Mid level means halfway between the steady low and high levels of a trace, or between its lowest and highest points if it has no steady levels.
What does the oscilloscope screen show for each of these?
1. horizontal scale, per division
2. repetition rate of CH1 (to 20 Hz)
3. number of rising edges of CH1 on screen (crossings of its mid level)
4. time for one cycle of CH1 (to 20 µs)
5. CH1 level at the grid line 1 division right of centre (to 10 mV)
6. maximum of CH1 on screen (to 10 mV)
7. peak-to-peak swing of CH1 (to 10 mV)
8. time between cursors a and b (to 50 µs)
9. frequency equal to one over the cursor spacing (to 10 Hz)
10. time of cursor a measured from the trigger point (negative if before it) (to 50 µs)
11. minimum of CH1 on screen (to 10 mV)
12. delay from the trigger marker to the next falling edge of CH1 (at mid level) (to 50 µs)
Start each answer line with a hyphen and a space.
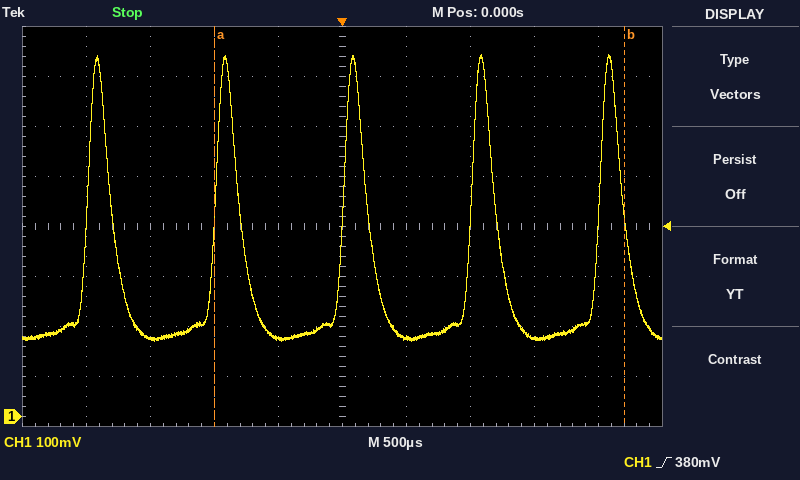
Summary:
- 500 µs
- 1.00 kHz
- 5
- 1.00 ms
- 160 mV
- 720 mV
- 570 mV
- 3.20 ms
- 310 Hz
- -1.00 ms
- 150 mV
- 200 µs
